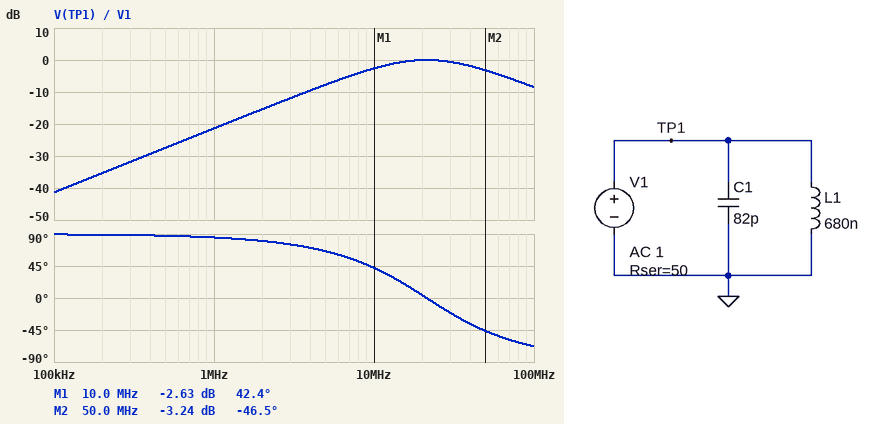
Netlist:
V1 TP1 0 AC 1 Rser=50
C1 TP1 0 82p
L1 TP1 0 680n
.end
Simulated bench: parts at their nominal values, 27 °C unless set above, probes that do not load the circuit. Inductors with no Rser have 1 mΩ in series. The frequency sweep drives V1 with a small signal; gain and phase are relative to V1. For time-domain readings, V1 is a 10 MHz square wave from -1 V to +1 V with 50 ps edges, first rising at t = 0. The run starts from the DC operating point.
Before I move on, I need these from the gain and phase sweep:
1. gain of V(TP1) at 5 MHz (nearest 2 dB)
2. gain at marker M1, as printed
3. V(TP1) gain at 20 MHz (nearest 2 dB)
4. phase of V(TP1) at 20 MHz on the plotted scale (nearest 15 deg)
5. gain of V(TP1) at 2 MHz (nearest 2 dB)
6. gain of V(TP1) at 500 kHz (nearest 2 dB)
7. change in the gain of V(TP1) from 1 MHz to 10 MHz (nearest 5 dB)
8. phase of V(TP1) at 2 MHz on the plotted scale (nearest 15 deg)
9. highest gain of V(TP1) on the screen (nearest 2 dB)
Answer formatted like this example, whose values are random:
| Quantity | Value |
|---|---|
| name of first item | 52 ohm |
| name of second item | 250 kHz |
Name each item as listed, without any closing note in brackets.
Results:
| Quantity | Value |
|---|---|
| gain of V(TP1) at 5 MHz | -8 dB |
| gain at marker M1, as printed | -2.63 dB |
| V(TP1) gain at 20 MHz | 0 dB |
| phase of V(TP1) at 20 MHz on the plotted scale | 0 deg |
| gain of V(TP1) at 2 MHz | -16 dB |
| gain of V(TP1) at 500 kHz | -28 dB |
| change in the gain of V(TP1) from 1 MHz to 10 MHz | 20 dB |
| phase of V(TP1) at 2 MHz on the plotted scale | 75 deg |
| highest gain of V(TP1) on the screen | 0 dB |
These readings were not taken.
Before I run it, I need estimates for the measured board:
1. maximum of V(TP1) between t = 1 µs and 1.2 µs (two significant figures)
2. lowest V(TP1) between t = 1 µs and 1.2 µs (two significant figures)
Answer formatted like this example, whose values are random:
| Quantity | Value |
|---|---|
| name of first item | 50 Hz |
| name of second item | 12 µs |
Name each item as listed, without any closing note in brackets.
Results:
| Quantity | Value |
|---|---|
| maximum of V(TP1) between t = 1 µs and 1.2 µs | 1.4 V |
| lowest V(TP1) between t = 1 µs and 1.2 µs | -1.4 V |
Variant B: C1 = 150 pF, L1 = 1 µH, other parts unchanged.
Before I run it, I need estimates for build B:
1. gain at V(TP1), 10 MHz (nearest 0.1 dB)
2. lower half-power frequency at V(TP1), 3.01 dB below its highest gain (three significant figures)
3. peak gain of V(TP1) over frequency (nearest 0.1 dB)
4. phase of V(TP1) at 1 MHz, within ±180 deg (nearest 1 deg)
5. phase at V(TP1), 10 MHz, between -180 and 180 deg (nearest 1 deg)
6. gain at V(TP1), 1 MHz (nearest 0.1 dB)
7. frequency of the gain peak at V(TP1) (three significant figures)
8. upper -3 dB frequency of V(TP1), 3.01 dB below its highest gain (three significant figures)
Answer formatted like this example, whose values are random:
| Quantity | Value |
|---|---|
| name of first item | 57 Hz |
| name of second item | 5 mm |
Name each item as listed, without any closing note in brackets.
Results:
| Quantity | Value |
|---|---|
| gain at V(TP1), 10 MHz | -0.4 dB |
| lower half-power frequency at V(TP1), 3.01 dB below its highest gain | 6.17 MHz |
| peak gain of V(TP1) over frequency | 0 dB |
| phase of V(TP1) at 1 MHz, within ±180 deg | 83 deg |
| phase at V(TP1), 10 MHz, between -180 and 180 deg | 18 deg |
| gain at V(TP1), 1 MHz | -18.0 dB |
| frequency of the gain peak at V(TP1) | 13.0 MHz |
| upper -3 dB frequency of V(TP1), 3.01 dB below its highest gain | 27.4 MHz |
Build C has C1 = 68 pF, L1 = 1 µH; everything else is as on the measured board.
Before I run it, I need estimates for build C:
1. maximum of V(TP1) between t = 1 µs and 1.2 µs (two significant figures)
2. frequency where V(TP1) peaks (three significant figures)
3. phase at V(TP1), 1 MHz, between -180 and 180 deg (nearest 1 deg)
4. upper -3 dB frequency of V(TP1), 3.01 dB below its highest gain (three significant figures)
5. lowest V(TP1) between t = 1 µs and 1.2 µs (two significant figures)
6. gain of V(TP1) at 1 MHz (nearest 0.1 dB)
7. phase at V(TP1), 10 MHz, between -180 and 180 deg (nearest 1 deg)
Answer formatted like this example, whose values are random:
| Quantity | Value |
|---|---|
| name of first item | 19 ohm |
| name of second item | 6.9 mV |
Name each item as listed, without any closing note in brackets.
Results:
| Quantity | Value |
|---|---|
| maximum of V(TP1) between t = 1 µs and 1.2 µs | 1.5 V |
| frequency where V(TP1) peaks | 19.3 MHz |
| phase at V(TP1), 1 MHz, between -180 and 180 deg | 83 deg |
| upper -3 dB frequency of V(TP1), 3.01 dB below its highest gain | 53.7 MHz |
| lowest V(TP1) between t = 1 µs and 1.2 µs | -1.5 V |
| gain of V(TP1) at 1 MHz | -18.1 dB |
| phase at V(TP1), 10 MHz, between -180 and 180 deg | 30 deg |
